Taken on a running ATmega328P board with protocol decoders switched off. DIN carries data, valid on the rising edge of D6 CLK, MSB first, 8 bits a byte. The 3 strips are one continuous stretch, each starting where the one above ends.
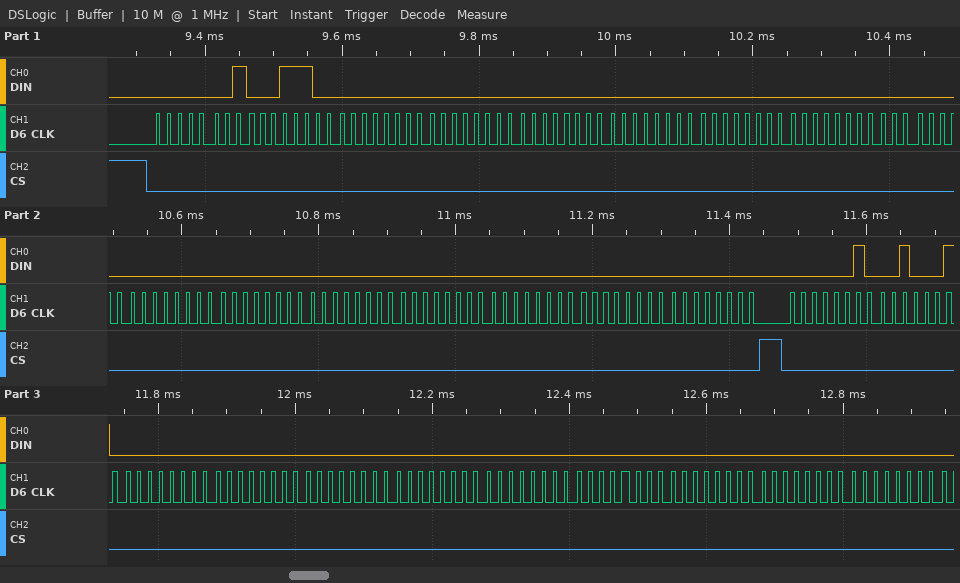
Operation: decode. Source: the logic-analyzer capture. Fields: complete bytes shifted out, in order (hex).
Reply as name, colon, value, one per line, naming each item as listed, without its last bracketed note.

complete bytes shifted out, in order: 01 1C 00 00 00 00 00 00 00 00 00 00 00 00 00 00 02 22 00 00 00 00 00 00 00 00 00
